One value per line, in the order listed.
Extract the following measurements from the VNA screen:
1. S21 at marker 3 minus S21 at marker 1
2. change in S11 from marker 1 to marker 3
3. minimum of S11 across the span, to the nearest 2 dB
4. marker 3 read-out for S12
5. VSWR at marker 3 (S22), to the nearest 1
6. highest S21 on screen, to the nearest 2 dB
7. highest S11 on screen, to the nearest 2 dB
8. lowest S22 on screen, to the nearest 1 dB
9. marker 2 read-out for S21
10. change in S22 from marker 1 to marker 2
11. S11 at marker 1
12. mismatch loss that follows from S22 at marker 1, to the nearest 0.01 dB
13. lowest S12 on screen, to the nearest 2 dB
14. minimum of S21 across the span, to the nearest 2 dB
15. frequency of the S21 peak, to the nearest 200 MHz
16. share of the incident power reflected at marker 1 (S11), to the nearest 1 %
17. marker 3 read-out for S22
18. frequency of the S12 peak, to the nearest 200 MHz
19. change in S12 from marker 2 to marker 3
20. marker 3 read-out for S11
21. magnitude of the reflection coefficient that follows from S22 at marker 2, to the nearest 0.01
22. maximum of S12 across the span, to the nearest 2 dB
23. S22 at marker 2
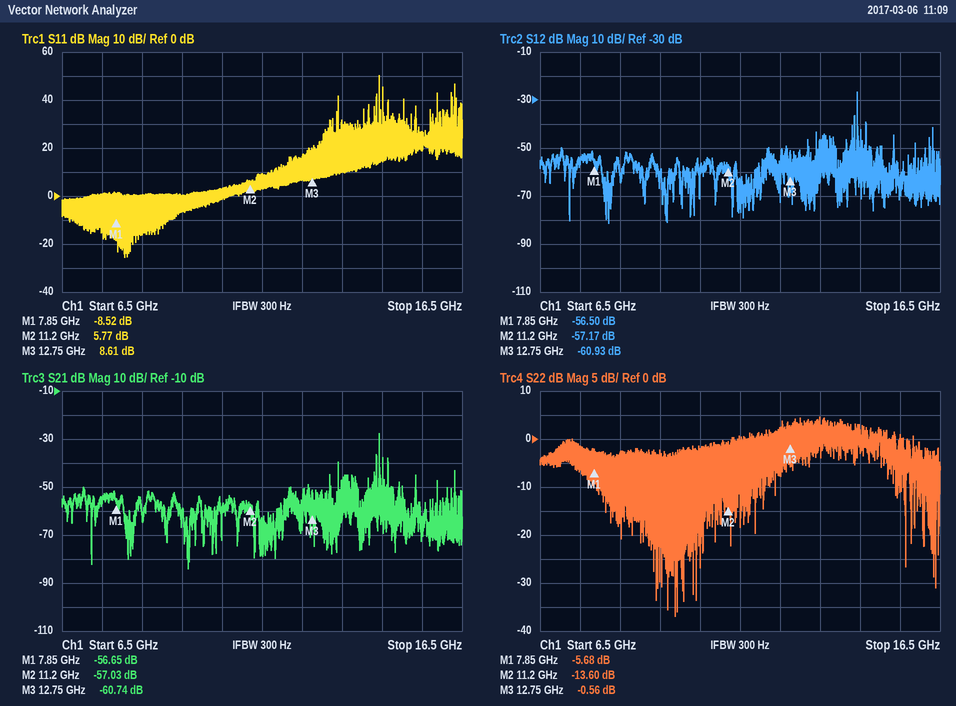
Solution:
-4.09 dB
17.13 dB
-26 dB
-60.93 dB
31
-28 dB
50 dB
-37 dB
-57.03 dB
-7.92 dB
-8.52 dB
1.37 dB
-82 dB
-84 dB
14.4 GHz
14 %
-0.56 dB
14.4 GHz
-3.76 dB
8.61 dB
0.21
-26 dB
-13.60 dB
